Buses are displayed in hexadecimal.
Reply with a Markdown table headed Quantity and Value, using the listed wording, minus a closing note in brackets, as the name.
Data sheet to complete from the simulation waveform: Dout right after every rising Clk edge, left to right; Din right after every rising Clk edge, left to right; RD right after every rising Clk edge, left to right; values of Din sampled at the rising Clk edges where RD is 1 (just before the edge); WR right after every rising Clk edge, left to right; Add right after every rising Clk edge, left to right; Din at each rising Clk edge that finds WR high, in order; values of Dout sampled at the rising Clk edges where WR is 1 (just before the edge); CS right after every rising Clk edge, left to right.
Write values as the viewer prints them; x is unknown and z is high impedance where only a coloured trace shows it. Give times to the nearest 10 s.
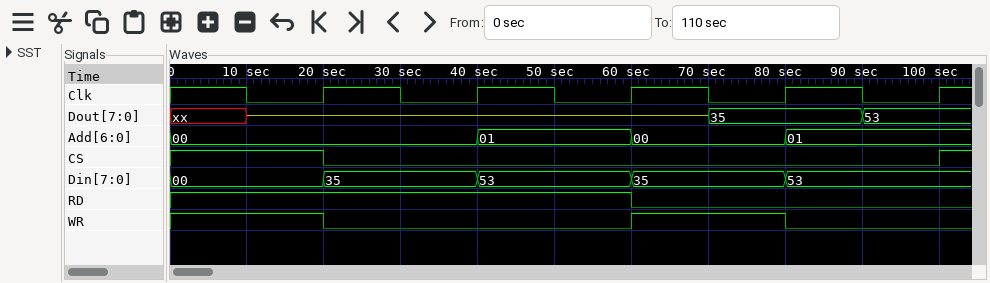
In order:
| Quantity | Value |
|---|---|
| Dout right after every rising Clk edge, left to right | z, z, z, 35, 53 |
| Din right after every rising Clk edge, left to right | 35, 53, 35, 53, 53 |
| RD right after every rising Clk edge, left to right | 1 1 0 0 0 |
| values of Din sampled at the rising Clk edges where RD is 1 | 00, 35, 53 |
| WR right after every rising Clk edge, left to right | 0 0 1 0 0 |
| Add right after every rising Clk edge, left to right | 00, 01, 00, 01, 01 |
| Din at each rising Clk edge that finds WR high, in order | 00, 35 |
| values of Dout sampled at the rising Clk edges where WR is 1 | z, 35 |
| CS right after every rising Clk edge, left to right | 0 0 0 0 1 |
